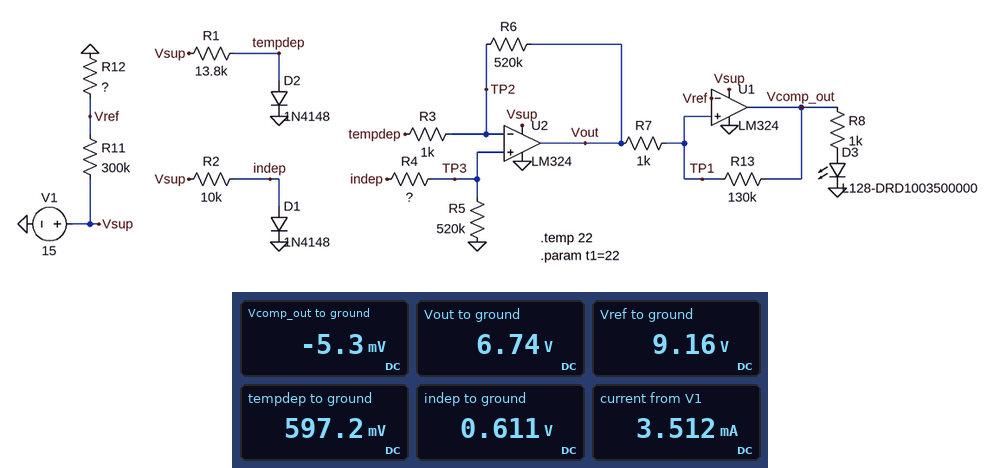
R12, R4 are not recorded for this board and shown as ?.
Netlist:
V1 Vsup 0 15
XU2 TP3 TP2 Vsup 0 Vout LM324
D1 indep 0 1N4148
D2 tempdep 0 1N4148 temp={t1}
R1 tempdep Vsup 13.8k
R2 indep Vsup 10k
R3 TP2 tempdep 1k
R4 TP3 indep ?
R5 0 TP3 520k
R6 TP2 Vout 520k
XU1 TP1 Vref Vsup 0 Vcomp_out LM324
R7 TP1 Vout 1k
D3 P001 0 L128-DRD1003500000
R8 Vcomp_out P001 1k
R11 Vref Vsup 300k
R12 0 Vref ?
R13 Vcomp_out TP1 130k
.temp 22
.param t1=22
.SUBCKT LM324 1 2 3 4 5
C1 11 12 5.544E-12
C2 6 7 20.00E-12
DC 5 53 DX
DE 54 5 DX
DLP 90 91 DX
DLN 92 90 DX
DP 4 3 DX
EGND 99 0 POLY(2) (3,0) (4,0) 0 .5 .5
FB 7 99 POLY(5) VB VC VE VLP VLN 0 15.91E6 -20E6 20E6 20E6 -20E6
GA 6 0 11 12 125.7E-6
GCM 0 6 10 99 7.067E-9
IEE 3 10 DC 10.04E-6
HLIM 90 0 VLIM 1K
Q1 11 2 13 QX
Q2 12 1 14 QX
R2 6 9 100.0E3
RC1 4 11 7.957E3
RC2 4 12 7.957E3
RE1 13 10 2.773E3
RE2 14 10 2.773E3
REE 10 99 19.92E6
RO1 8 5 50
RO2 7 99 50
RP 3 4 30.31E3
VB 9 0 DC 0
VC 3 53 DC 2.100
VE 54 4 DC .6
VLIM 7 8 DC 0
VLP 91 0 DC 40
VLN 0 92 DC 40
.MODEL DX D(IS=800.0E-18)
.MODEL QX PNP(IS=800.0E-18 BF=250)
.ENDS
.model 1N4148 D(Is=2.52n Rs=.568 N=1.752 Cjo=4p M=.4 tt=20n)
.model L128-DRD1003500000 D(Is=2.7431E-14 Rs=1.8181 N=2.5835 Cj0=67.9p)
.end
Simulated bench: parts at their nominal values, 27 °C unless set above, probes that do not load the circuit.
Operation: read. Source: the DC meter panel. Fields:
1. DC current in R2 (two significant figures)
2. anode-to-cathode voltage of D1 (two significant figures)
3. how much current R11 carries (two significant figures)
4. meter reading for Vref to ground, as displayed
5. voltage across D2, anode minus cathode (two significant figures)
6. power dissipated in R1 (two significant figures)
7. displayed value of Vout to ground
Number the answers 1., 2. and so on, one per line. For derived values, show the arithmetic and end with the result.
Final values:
1. (15 V - 611 mV) / 10 kΩ = 1.4 mA
2. 611 mV = 610 mV
3. (15 V - 9.16 V) / 300 kΩ = 19 µA
4. 9.16 V
5. 597.2 mV = 600 mV
6. (15 V - 597.2 mV)^2 / 13.8 kΩ = 15 mW
7. 6.74 V
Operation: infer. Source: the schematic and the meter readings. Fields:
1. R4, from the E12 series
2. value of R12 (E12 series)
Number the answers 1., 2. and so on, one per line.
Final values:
1. 2.2 kΩ
2. 470 kΩ
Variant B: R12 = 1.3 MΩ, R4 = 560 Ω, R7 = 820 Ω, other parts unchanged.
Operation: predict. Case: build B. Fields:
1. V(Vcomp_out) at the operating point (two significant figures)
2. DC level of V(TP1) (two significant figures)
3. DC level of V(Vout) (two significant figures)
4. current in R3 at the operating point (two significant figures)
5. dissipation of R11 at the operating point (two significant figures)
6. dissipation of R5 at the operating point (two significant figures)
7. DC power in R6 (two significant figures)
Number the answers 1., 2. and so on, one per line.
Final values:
1. -5.2 mV
2. 7.6 V
3. 7.7 V
4. 14 µA
5. 26 µW
6. 720 nW
7. 96 µW
